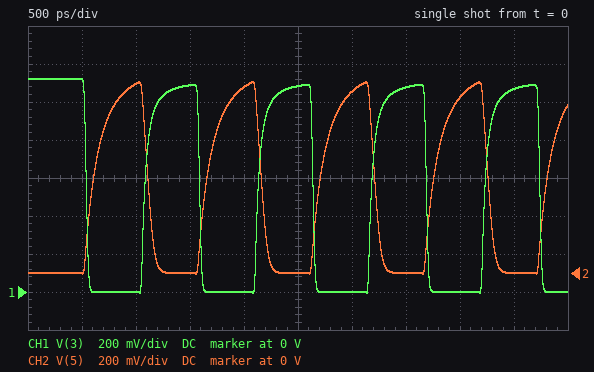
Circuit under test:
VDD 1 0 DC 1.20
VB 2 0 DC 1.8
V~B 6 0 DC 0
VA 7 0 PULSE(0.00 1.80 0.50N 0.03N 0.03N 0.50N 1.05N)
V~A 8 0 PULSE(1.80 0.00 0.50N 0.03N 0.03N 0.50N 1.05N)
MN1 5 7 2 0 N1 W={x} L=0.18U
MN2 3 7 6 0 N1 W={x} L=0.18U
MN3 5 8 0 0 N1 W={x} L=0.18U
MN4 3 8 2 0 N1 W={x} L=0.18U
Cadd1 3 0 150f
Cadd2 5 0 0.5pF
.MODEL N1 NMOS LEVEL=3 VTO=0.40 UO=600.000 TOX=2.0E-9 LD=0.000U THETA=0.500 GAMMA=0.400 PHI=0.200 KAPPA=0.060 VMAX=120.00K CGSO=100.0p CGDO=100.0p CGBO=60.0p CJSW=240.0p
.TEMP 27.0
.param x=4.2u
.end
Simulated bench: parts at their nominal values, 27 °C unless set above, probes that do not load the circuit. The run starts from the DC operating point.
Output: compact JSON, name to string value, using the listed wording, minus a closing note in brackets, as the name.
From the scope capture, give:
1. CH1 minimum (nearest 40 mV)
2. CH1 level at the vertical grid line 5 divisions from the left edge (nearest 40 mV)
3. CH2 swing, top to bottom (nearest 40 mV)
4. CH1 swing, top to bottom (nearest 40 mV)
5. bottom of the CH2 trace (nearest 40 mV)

{"CH1 minimum": "0 V", "CH1 level at the vertical grid line 5 divisions from the left edge": "1.08 V", "CH2 swing, top to bottom": "1.00 V", "CH1 swing, top to bottom": "1.12 V", "bottom of the CH2 trace": "0 V"}
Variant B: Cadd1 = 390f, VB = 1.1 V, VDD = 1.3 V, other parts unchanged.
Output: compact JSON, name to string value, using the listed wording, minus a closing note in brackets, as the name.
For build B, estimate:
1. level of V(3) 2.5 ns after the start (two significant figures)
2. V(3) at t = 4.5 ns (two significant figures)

{"level of V(3) 2.5 ns after the start": "1.0 V", "V(3) at t = 4.5 ns": "960 mV"}
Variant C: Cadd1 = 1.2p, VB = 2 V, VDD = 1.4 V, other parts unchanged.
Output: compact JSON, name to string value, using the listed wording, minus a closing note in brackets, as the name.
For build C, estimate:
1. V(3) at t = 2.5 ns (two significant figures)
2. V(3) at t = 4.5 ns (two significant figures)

{"V(3) at t = 2.5 ns": "730 mV", "V(3) at t = 4.5 ns": "630 mV"}
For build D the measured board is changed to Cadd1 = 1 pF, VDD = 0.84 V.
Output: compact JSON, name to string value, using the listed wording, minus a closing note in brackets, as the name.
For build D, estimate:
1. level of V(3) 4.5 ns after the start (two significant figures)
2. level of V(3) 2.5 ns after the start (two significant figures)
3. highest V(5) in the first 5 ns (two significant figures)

{"level of V(3) 4.5 ns after the start": "690 mV", "level of V(3) 2.5 ns after the start": "790 mV", "highest V(5) in the first 5 ns": "1.0 V"}
